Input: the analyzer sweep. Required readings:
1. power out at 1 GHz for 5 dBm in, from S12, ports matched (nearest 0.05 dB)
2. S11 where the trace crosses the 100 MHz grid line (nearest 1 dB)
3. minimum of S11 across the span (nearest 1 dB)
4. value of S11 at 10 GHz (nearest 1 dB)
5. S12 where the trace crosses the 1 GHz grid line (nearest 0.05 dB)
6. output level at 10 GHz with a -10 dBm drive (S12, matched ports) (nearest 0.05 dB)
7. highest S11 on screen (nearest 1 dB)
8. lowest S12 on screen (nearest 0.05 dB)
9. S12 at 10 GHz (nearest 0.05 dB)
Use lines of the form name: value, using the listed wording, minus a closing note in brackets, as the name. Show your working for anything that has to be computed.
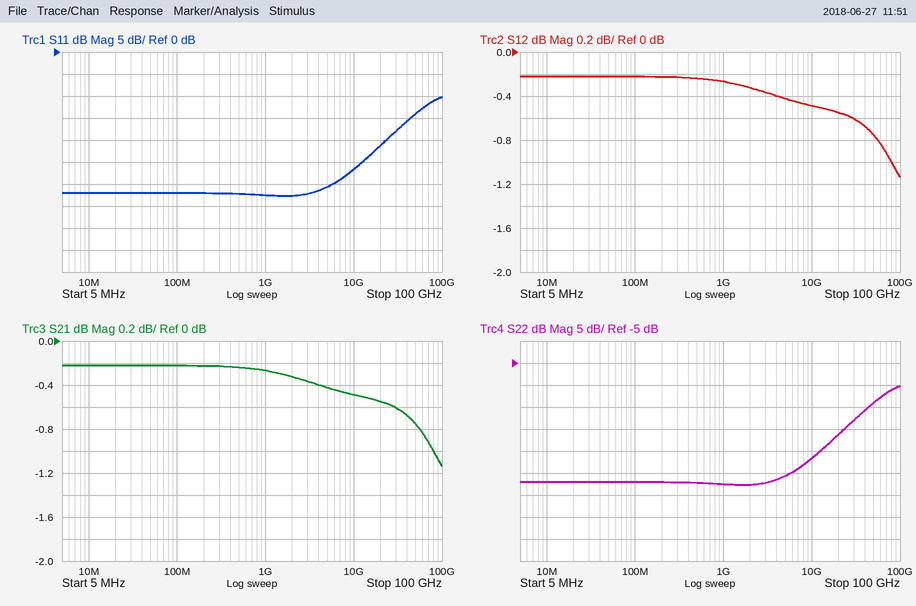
power out at 1 GHz for 5 dBm in, from S12, ports matched: 5 dBm + (-0.25 dB) = 4.75 dBm
S11 where the trace crosses the 100 MHz grid line: -32 dB
minimum of S11 across the span: -33 dB
value of S11 at 10 GHz: -27 dB
S12 where the trace crosses the 1 GHz grid line: -0.25 dB
output level at 10 GHz with a -10 dBm drive (S12, matched ports): -10 dBm + (-0.50 dB) = -10.50 dBm
highest S11 on screen: -10 dB
lowest S12 on screen: -1.15 dB
S12 at 10 GHz: -0.50 dB
